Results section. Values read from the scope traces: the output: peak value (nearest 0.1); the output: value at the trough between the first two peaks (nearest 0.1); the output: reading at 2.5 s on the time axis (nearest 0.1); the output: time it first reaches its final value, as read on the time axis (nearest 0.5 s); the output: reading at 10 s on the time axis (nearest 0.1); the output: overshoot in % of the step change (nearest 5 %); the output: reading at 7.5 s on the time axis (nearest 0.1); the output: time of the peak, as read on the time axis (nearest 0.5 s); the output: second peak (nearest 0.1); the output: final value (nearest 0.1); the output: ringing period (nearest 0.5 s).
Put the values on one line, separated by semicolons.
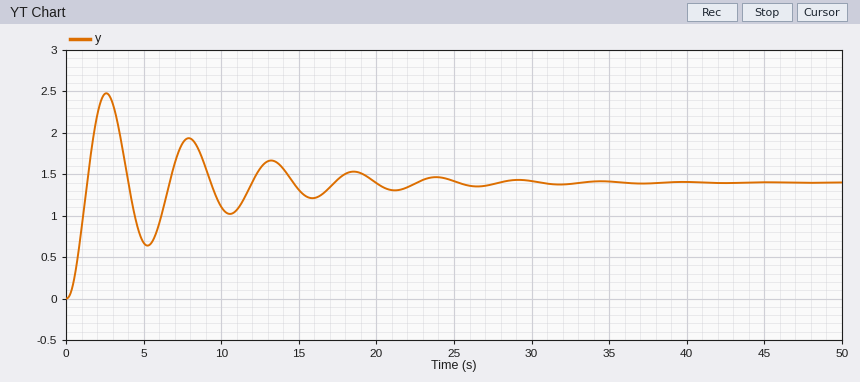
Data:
2.5; 0.6; 2.5; 1.5 s; 1.1; 75 %; 1.9; 2.5 s; 1.9; 1.4; 5.5 s
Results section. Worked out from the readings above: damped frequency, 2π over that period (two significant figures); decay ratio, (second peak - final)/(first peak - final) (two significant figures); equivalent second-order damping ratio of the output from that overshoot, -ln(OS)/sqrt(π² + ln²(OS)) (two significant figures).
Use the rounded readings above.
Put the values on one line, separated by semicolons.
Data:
1.1 rad/s; 0.45; 0.091
